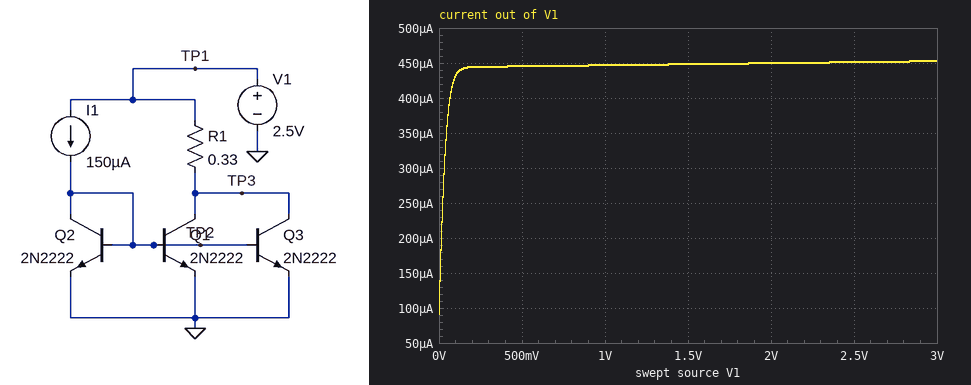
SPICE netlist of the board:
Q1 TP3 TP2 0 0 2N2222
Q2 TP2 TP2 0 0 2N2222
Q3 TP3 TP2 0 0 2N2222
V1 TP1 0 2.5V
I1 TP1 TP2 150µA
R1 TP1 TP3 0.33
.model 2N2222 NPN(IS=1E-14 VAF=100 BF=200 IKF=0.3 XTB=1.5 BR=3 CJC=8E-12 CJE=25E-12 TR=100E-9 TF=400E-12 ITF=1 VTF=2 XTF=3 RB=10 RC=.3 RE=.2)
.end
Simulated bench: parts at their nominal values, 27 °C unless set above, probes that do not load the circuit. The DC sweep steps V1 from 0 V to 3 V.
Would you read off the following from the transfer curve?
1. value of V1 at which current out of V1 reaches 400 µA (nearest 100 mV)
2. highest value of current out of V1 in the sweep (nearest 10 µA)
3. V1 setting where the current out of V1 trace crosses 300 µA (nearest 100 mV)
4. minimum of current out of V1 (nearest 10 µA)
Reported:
100 mV
450 µA
0 V
90 µA
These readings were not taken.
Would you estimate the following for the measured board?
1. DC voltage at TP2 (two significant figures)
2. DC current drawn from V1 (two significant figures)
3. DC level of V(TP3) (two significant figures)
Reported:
610 mV
450 µA
2.5 V
